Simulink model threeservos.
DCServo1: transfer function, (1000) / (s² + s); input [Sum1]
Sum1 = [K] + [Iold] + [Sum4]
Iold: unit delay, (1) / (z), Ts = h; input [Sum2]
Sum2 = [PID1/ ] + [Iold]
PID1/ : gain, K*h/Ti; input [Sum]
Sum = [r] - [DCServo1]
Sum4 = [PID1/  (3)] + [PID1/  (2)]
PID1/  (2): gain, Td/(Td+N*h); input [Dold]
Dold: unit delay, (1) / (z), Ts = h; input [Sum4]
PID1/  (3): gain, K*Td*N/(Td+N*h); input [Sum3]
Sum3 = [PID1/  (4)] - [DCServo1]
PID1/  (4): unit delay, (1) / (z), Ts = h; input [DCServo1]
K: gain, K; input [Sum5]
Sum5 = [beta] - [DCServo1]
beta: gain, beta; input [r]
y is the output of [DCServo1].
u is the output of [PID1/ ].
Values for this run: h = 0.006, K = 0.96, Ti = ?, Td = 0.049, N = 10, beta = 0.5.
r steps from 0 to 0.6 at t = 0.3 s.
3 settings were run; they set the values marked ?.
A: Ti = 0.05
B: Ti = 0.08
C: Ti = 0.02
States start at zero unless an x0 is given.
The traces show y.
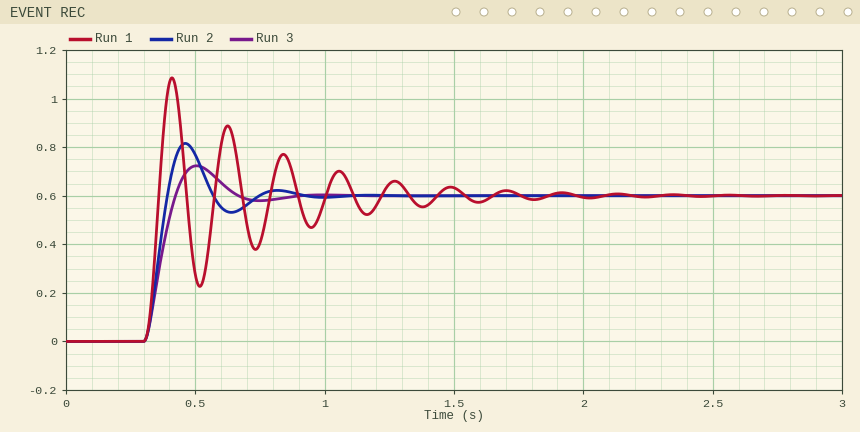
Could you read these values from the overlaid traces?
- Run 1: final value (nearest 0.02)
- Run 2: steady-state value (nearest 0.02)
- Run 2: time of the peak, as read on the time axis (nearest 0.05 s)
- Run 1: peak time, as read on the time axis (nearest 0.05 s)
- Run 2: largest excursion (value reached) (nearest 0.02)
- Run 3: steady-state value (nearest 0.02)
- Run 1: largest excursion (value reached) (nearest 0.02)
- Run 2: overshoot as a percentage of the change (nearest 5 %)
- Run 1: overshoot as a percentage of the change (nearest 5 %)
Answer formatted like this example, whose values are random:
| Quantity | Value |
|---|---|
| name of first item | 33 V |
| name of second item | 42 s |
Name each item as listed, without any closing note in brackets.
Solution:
| Quantity | Value |
|---|---|
| Run 1: final value | 0.60 |
| Run 2: steady-state value | 0.60 |
| Run 2: time of the peak, as read on the time axis | 0.45 s |
| Run 1: peak time, as read on the time axis | 0.40 s |
| Run 2: largest excursion (value reached) | 0.82 |
| Run 3: steady-state value | 0.60 |
| Run 1: largest excursion (value reached) | 1.08 |
| Run 2: overshoot as a percentage of the change | 35 % |
| Run 1: overshoot as a percentage of the change | 80 % |
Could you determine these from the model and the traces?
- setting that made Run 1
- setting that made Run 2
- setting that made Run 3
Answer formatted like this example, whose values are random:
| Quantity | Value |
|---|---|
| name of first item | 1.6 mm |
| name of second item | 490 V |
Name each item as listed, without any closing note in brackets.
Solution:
| Quantity | Value |
|---|---|
| setting that made Run 1 | C |
| setting that made Run 2 | A |
| setting that made Run 3 | B |
